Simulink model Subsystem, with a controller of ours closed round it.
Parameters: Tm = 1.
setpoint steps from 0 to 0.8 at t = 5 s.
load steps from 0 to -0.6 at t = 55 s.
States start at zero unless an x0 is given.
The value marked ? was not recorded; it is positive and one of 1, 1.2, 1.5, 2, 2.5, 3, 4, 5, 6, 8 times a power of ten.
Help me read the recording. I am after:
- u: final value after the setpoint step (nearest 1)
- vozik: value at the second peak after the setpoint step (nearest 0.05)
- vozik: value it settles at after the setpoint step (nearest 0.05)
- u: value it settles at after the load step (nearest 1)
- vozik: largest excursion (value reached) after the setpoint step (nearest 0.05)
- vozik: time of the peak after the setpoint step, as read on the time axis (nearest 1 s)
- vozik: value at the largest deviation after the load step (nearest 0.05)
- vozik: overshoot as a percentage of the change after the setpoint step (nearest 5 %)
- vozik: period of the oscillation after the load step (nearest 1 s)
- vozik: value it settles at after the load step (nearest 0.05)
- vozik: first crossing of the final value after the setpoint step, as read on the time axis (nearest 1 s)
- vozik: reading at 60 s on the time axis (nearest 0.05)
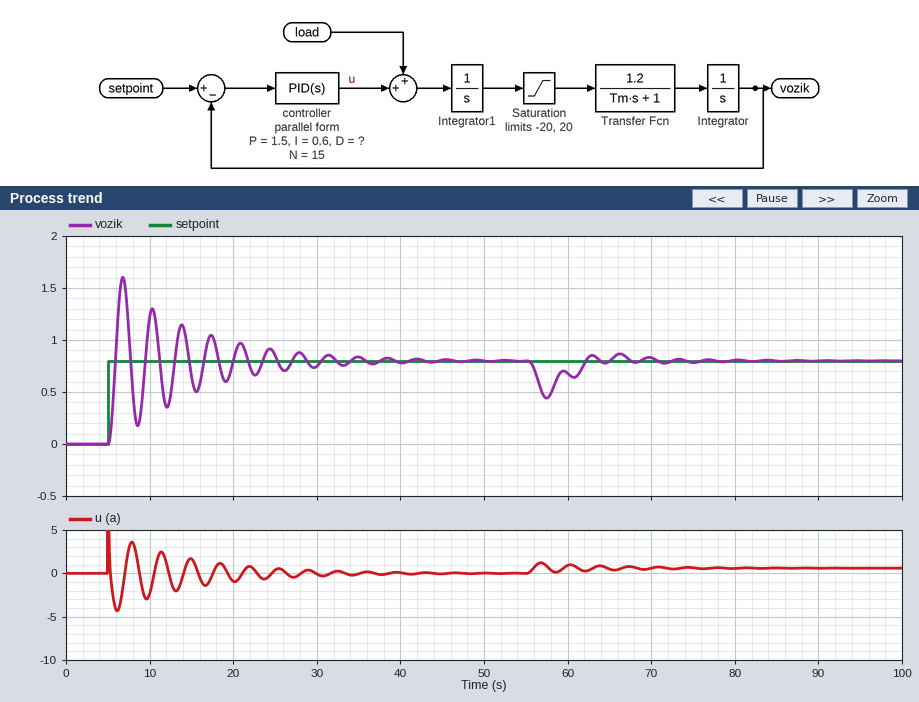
0
1.30
0.80
1
1.60
7 s
0.45
100 %
3 s
0.80
6 s
0.70
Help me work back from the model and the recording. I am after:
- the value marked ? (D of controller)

3
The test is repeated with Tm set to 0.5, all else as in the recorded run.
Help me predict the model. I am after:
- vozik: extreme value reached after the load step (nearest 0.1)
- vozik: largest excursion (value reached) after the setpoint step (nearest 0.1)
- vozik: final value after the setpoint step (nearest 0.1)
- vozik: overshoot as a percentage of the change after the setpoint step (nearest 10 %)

0.5
1.4
0.8
70 %
